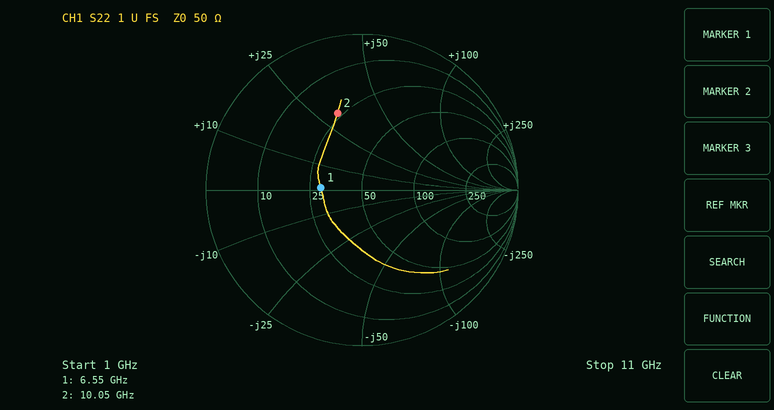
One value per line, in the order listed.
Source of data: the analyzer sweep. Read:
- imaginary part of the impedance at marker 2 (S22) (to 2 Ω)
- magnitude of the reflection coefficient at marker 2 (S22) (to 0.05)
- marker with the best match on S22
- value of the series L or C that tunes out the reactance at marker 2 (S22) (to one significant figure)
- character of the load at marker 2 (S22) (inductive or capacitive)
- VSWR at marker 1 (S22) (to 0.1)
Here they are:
+32 Ω
0.50
marker 1
500 fF
inductive
1.7
